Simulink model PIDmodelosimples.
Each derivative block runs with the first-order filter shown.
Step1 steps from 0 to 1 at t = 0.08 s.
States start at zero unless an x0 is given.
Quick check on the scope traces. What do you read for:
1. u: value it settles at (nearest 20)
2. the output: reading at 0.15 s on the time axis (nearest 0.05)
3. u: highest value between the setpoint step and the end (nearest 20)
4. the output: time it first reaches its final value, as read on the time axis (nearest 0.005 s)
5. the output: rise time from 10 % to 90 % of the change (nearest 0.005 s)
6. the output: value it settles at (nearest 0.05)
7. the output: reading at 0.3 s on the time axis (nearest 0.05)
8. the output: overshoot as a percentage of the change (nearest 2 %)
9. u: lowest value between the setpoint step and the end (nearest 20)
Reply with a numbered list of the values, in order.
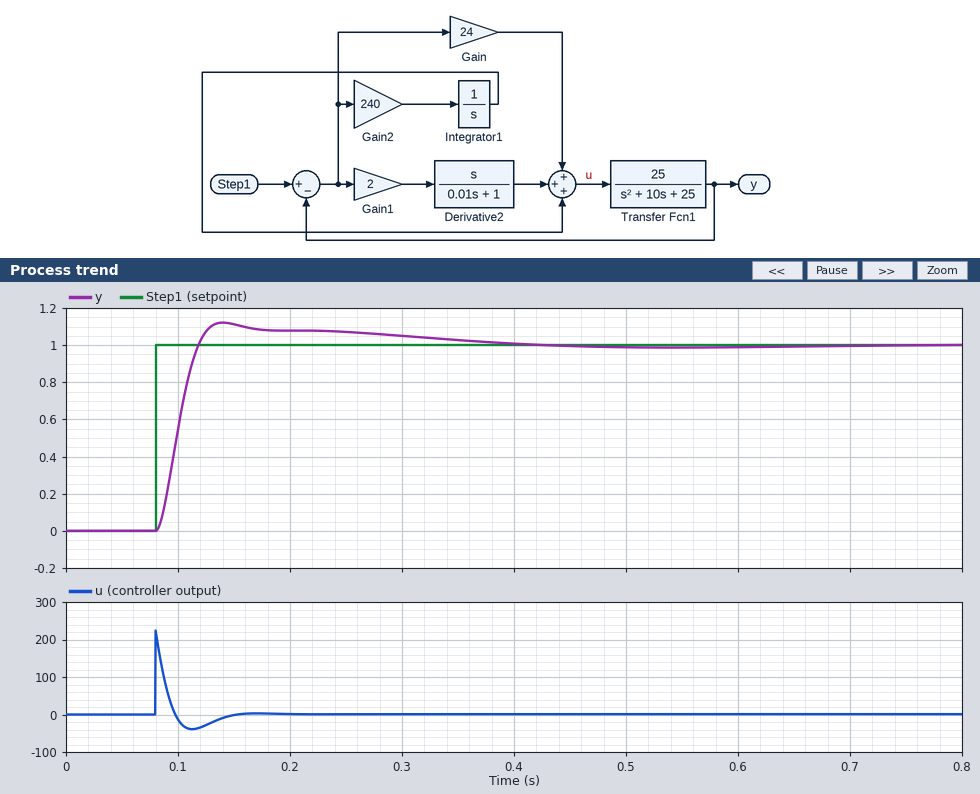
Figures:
1. 0
2. 1.10
3. 220
4. 0.120 s
5. 0.025 s
6. 1.00
7. 1.05
8. 12 %
9. -40
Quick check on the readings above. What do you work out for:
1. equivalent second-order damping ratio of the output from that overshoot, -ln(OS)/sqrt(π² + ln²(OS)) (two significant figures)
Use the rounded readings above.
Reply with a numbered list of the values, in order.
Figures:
1. 0.56
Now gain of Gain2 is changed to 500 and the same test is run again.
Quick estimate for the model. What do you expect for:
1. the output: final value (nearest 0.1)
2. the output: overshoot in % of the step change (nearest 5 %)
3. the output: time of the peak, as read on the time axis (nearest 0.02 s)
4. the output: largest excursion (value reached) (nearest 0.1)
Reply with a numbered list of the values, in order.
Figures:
1. 1.0
2. 20 %
3. 0.14 s
4. 1.2
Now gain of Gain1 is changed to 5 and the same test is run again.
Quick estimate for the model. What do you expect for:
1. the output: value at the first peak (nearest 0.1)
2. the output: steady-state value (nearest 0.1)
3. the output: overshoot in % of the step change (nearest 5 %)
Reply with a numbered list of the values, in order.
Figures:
1. 1.2
2. 1.0
3. 15 %
